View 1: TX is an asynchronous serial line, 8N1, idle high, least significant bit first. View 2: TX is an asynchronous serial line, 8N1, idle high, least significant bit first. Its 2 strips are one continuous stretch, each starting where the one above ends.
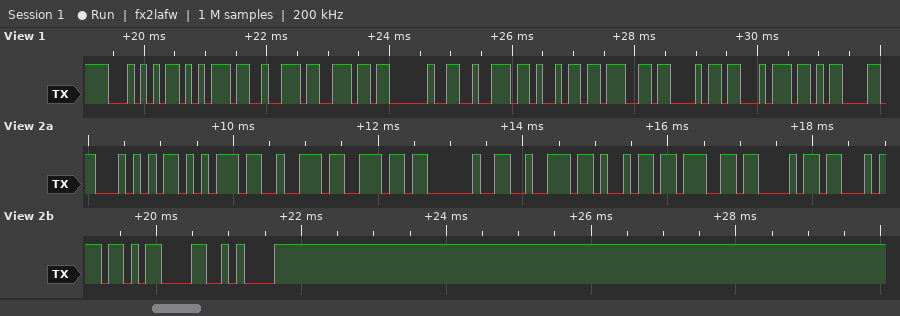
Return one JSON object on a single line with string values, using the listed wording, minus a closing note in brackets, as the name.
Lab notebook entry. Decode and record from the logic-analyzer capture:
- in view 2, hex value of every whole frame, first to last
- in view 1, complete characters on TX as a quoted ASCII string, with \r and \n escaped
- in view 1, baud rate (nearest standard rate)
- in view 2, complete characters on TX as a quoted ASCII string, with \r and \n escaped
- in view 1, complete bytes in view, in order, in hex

{"in view 2, hex value of every whole frame, first to last": "0x54 0x75 0x72 0x6E 0x20 0x72 0x69 0x67 0x68 0x74 0x0D 0x0A", "in view 1, complete characters on TX as a quoted ASCII string, with \\r and \\n escaped": "\"Turn right\\r\"", "in view 1, baud rate": "9600 baud", "in view 2, complete characters on TX as a quoted ASCII string, with \\r and \\n escaped": "\"Turn right\\r\\n\"", "in view 1, complete bytes in view, in order, in hex": "0x54 0x75 0x72 0x6E 0x20 0x72 0x69 0x67 0x68 0x74 0x0D"}
